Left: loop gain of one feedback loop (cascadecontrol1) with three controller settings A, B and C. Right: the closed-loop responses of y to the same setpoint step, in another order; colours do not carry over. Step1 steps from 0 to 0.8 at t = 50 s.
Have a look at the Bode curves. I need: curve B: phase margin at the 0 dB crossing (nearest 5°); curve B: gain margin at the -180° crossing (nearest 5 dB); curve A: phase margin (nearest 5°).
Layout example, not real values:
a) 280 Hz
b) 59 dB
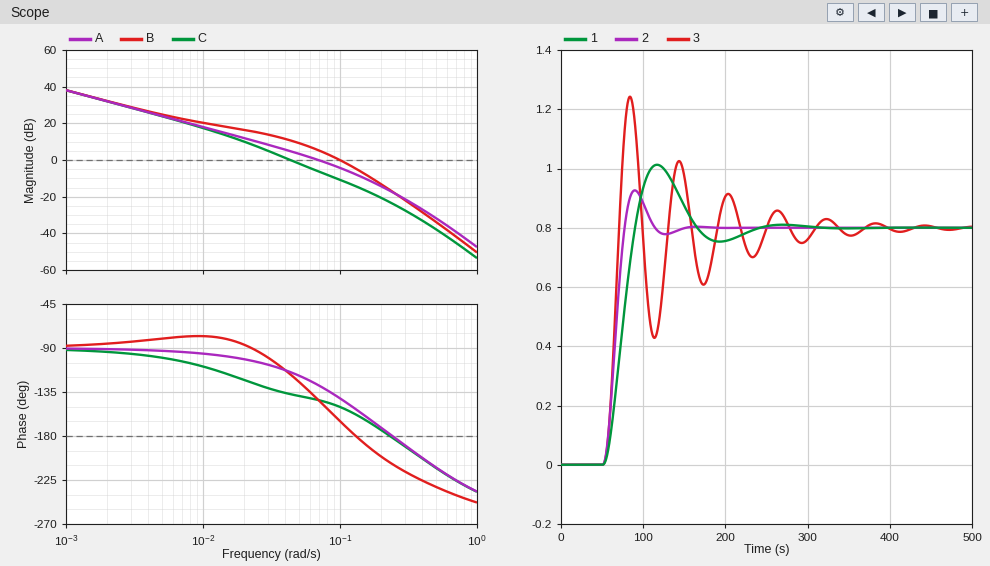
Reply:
a) 15°
b) 5 dB
c) 50°
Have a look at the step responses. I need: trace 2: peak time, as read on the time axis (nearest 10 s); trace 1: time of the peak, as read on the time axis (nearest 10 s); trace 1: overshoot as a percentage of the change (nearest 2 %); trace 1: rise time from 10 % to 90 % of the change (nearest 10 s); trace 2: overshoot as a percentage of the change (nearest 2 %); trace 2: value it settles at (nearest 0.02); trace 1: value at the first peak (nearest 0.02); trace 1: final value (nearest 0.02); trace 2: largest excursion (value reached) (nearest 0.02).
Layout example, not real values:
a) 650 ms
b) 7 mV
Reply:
a) 90 s
b) 120 s
c) 26 %
d) 30 s
e) 16 %
f) 0.80
g) 1.02
h) 0.80
i) 0.92
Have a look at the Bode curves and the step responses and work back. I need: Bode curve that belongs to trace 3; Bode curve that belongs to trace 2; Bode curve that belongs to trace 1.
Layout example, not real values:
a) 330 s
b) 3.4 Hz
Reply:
a) B
b) A
c) C
